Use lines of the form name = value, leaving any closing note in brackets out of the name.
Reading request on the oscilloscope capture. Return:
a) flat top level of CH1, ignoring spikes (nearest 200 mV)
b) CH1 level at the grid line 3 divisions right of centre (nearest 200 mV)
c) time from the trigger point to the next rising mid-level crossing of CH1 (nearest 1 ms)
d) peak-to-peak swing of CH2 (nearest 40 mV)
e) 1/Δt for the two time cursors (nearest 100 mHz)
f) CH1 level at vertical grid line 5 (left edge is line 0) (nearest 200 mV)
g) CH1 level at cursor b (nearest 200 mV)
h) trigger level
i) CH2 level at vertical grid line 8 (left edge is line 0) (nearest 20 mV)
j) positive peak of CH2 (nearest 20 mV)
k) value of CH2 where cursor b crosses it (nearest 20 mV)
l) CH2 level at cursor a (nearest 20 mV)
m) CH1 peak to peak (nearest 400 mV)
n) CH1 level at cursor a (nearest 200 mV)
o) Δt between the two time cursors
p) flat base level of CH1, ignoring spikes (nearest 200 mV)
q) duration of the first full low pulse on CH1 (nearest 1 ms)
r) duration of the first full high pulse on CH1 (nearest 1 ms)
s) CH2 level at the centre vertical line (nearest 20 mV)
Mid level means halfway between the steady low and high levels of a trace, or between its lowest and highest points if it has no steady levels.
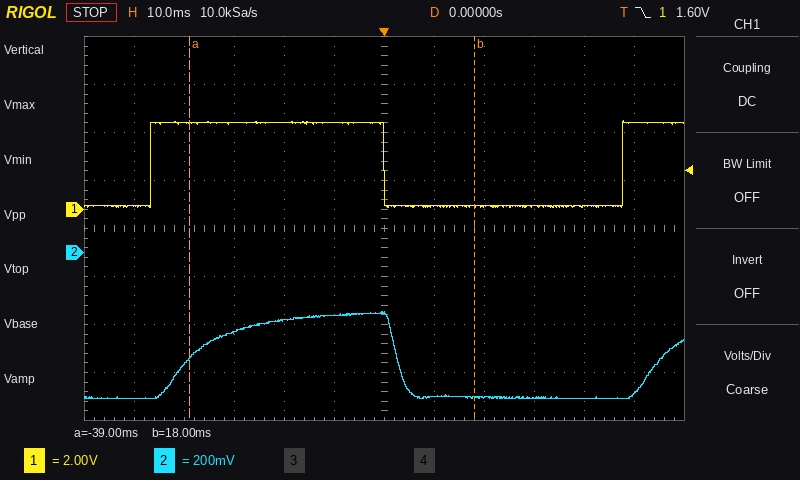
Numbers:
flat top level of CH1, ignoring spikes = 3.6 V
CH1 level at the grid line 3 divisions right of centre = 200 mV
time from the trigger point to the next rising mid-level crossing of CH1 = 48 ms
peak-to-peak swing of CH2 = 360 mV
1/Δt for the two time cursors = 17.5 Hz
CH1 level at vertical grid line 5 (left edge is line 0) = 3.6 V
CH1 level at cursor b = 200 mV
trigger level = 1.60 V
CH2 level at vertical grid line 8 (left edge is line 0) = -600 mV
positive peak of CH2 = -240 mV
value of CH2 where cursor b crosses it = -600 mV
CH2 level at cursor a = -440 mV
CH1 peak to peak = 3.6 V
CH1 level at cursor a = 3.6 V
Δt between the two time cursors = 57 ms
flat base level of CH1, ignoring spikes = 200 mV
duration of the first full low pulse on CH1 = 48 ms
duration of the first full high pulse on CH1 = 47 ms
CH2 level at the centre vertical line = -260 mV
